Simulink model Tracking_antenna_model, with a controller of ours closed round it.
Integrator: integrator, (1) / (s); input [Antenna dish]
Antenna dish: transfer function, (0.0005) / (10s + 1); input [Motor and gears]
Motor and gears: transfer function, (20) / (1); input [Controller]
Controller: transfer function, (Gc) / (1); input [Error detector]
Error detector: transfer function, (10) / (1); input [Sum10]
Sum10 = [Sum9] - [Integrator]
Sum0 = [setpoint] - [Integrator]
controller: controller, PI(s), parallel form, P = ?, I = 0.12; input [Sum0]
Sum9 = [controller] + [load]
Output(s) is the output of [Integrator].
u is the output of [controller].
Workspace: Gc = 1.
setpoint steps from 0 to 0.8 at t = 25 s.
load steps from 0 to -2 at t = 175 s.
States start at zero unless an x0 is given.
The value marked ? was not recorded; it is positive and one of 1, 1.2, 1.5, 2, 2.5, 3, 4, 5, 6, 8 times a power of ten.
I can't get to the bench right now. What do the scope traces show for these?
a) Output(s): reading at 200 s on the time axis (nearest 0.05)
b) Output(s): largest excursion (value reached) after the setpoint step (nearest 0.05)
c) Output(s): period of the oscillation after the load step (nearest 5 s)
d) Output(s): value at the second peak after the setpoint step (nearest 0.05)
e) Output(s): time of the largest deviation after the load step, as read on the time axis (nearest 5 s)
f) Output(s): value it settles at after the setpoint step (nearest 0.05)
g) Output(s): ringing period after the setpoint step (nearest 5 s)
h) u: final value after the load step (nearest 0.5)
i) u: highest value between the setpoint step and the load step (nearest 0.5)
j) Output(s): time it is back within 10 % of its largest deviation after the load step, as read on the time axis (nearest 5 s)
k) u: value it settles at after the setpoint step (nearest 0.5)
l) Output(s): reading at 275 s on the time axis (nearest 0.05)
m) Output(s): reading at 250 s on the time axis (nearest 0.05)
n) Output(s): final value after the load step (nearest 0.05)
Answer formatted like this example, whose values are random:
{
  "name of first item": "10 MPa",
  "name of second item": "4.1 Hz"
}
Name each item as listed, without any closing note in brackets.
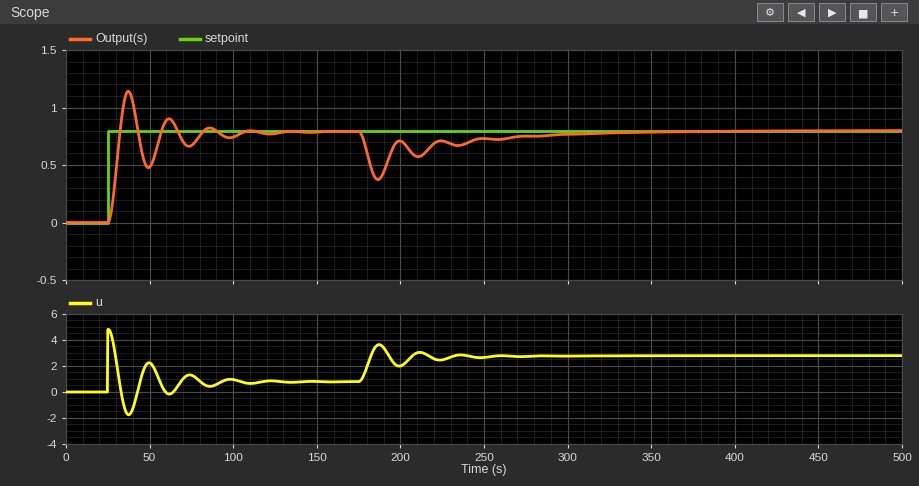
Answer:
{
  "Output(s): reading at 200 s on the time axis": "0.70",
  "Output(s): largest excursion (value reached) after the setpoint step": "1.15",
  "Output(s): period of the oscillation after the load step": "25 s",
  "Output(s): value at the second peak after the setpoint step": "0.90",
  "Output(s): time of the largest deviation after the load step, as read on the time axis": "185 s",
  "Output(s): value it settles at after the setpoint step": "0.80",
  "Output(s): ringing period after the setpoint step": "25 s",
  "u: final value after the load step": "3.0",
  "u: highest value between the setpoint step and the load step": "5.0",
  "Output(s): time it is back within 10 % of its largest deviation after the load step, as read on the time axis": "290 s",
  "u: value it settles at after the setpoint step": "1.0",
  "Output(s): reading at 275 s on the time axis": "0.75",
  "Output(s): reading at 250 s on the time axis": "0.75",
  "Output(s): final value after the load step": "0.80"
}
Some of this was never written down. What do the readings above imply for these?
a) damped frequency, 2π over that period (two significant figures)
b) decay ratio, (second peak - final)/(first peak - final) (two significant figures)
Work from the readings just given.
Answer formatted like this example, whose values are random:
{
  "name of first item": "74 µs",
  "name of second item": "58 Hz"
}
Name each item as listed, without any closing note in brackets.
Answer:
{
  "damped frequency, 2π over that period": "0.25 rad/s",
  "decay ratio, (second peak - final)/(first peak - final)": "0.29"
}
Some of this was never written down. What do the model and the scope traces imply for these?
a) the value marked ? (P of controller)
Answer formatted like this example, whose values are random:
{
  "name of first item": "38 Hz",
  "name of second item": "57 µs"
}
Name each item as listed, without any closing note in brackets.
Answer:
{
  "the value marked ?": "6"
}
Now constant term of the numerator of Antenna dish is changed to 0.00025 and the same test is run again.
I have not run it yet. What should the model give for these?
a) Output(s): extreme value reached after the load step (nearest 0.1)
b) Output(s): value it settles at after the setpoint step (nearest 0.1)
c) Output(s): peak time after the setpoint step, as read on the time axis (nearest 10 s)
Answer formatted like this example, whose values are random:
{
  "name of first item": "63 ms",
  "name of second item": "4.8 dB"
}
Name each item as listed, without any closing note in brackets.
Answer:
{
  "Output(s): extreme value reached after the load step": "0.4",
  "Output(s): value it settles at after the setpoint step": "0.8",
  "Output(s): peak time after the setpoint step, as read on the time axis": "40 s"
}
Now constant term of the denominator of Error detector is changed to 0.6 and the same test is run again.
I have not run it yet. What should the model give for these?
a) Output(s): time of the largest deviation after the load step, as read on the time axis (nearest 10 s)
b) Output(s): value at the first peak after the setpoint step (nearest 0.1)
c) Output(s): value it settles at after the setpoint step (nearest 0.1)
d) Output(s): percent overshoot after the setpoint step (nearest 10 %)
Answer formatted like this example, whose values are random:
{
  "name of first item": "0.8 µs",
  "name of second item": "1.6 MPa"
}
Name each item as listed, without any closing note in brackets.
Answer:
{
  "Output(s): time of the largest deviation after the load step, as read on the time axis": "180 s",
  "Output(s): value at the first peak after the setpoint step": "1.2",
  "Output(s): value it settles at after the setpoint step": "0.8",
  "Output(s): percent overshoot after the setpoint step": "50 %"
}
